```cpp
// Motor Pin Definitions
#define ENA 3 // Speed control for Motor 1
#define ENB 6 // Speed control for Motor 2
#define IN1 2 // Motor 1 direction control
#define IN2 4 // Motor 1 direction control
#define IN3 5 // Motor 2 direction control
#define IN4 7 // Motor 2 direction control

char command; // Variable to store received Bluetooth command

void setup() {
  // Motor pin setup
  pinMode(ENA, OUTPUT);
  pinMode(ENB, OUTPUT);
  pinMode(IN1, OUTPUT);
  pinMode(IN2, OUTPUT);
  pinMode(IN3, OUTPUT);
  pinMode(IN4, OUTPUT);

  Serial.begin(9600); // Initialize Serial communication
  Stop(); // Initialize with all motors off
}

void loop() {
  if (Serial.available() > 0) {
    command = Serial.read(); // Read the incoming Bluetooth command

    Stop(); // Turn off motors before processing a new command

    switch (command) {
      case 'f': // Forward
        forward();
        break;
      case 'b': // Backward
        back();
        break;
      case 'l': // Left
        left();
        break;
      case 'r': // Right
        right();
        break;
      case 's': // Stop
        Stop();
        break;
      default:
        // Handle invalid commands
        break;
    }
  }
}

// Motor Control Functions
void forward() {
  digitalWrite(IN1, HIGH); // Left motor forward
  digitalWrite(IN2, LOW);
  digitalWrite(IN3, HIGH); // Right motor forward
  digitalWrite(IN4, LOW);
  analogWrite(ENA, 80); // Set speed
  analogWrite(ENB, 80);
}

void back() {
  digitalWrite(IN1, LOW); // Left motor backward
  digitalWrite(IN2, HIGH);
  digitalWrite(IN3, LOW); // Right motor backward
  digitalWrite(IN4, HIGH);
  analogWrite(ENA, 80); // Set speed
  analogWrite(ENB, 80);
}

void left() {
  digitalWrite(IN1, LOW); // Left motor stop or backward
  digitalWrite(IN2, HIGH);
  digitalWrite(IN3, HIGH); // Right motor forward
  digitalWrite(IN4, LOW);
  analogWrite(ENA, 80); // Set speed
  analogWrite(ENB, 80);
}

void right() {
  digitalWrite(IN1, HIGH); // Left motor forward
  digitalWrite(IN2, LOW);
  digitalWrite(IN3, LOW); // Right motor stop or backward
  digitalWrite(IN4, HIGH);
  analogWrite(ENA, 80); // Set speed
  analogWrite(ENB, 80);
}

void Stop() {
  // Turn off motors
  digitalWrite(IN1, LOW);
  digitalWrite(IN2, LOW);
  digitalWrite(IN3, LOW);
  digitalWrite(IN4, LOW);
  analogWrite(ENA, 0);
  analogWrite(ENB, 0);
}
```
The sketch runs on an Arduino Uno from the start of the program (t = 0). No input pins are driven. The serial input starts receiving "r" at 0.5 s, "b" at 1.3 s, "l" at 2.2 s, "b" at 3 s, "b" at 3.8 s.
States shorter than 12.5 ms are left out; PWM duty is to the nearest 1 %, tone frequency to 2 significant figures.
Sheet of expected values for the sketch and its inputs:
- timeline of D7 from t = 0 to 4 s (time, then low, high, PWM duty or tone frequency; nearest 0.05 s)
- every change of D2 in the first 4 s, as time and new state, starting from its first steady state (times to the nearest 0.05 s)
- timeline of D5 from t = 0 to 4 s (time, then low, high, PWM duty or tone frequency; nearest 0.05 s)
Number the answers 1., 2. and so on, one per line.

1. 0 s low; 0.5 s high; 2.2 s low; 3 s high
2. 0 s low; 0.5 s high; 1.3 s low
3. 0 s low; 2.2 s high; 3 s low
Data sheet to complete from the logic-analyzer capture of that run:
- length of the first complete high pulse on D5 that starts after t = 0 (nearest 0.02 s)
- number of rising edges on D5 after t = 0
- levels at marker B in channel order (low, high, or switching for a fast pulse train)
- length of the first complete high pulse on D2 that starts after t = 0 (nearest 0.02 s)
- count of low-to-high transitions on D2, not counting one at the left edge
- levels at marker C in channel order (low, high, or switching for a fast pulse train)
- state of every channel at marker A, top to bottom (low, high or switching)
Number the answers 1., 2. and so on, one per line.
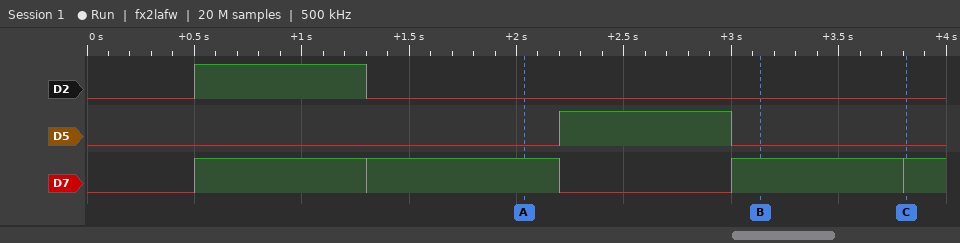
1. 0.80 s
2. 1
3. D2 low, D5 low, D7 high
4. 0.80 s
5. 1
6. D2 low, D5 low, D7 high
7. D2 low, D5 low, D7 high
